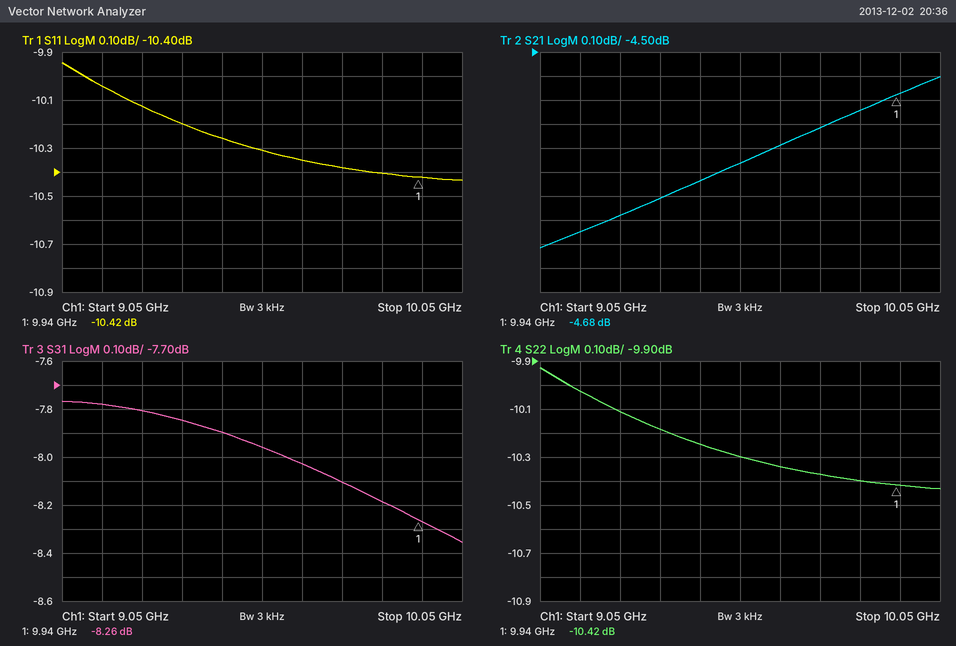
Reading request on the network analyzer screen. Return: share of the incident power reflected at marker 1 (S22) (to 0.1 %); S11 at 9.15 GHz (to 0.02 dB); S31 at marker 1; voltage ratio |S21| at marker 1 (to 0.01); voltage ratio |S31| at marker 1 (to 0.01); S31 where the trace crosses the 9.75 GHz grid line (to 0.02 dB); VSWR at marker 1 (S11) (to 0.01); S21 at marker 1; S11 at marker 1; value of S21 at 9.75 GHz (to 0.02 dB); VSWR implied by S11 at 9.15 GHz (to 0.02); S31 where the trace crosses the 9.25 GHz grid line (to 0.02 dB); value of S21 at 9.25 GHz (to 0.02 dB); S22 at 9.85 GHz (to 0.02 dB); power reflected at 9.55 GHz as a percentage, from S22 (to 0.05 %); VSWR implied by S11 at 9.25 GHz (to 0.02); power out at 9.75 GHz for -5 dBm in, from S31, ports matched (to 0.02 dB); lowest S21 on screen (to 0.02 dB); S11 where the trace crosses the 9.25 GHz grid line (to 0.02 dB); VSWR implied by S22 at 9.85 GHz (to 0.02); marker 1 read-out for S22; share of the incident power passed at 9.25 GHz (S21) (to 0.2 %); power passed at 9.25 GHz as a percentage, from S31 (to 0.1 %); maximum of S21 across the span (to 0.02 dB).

9.1 %
-10.04 dB
-8.26 dB
0.58
0.39
-8.10 dB
1.86
-4.68 dB
-10.42 dB
-4.82 dB
1.92
-7.80 dB
-5.18 dB
-10.40 dB
9.35 %
1.90
-13.10 dBm
-5.32 dB
-10.12 dB
1.86
-10.42 dB
30.4 %
16.6 %
-4.60 dB
